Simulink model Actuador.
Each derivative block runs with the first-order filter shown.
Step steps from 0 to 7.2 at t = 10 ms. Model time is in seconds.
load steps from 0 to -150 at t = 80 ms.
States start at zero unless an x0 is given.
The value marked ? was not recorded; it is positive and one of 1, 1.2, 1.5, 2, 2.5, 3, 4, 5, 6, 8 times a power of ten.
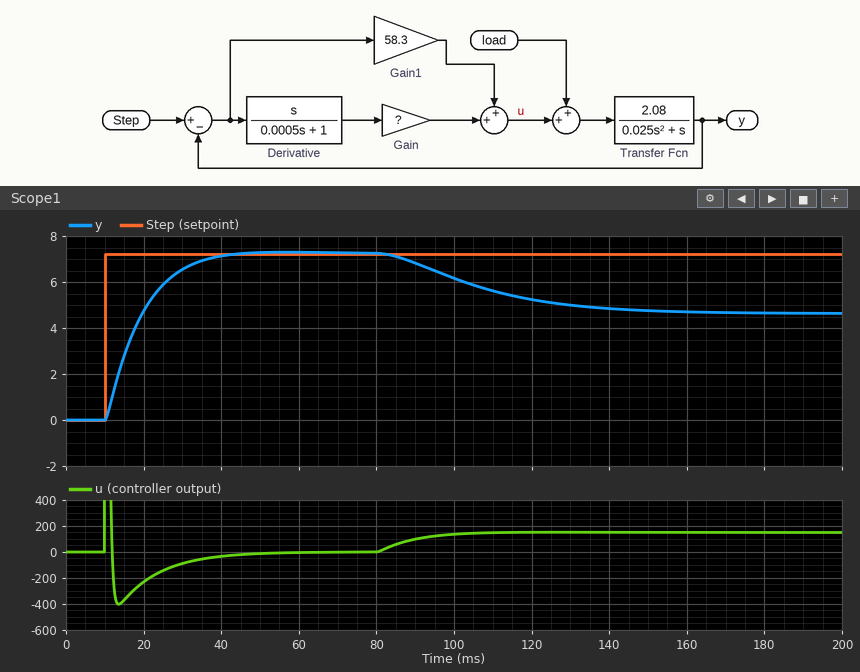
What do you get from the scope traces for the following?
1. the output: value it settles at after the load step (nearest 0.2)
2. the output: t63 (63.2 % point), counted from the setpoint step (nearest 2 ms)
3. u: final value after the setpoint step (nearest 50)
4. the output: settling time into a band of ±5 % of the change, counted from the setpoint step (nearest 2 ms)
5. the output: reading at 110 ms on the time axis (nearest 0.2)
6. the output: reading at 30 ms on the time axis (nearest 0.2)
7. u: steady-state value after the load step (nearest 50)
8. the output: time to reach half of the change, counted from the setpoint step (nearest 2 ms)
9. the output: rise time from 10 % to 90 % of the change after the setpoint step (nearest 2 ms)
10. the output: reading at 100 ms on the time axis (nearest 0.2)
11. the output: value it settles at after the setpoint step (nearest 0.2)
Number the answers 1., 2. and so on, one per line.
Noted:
1. 4.6
2. 10 ms
3. 0
4. 24 ms
5. 5.6
6. 6.6
7. 150
8. 6 ms
9. 18 ms
10. 6.2
11. 7.2
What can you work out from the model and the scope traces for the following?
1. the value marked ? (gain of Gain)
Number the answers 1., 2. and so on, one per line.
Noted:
1. 1.2
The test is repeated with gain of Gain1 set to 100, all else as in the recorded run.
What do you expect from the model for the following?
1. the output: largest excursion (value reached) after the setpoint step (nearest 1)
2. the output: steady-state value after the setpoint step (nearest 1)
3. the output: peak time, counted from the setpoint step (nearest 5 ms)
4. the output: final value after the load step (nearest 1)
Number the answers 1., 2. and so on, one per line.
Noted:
1. 8
2. 7
3. 30 ms
4. 6
